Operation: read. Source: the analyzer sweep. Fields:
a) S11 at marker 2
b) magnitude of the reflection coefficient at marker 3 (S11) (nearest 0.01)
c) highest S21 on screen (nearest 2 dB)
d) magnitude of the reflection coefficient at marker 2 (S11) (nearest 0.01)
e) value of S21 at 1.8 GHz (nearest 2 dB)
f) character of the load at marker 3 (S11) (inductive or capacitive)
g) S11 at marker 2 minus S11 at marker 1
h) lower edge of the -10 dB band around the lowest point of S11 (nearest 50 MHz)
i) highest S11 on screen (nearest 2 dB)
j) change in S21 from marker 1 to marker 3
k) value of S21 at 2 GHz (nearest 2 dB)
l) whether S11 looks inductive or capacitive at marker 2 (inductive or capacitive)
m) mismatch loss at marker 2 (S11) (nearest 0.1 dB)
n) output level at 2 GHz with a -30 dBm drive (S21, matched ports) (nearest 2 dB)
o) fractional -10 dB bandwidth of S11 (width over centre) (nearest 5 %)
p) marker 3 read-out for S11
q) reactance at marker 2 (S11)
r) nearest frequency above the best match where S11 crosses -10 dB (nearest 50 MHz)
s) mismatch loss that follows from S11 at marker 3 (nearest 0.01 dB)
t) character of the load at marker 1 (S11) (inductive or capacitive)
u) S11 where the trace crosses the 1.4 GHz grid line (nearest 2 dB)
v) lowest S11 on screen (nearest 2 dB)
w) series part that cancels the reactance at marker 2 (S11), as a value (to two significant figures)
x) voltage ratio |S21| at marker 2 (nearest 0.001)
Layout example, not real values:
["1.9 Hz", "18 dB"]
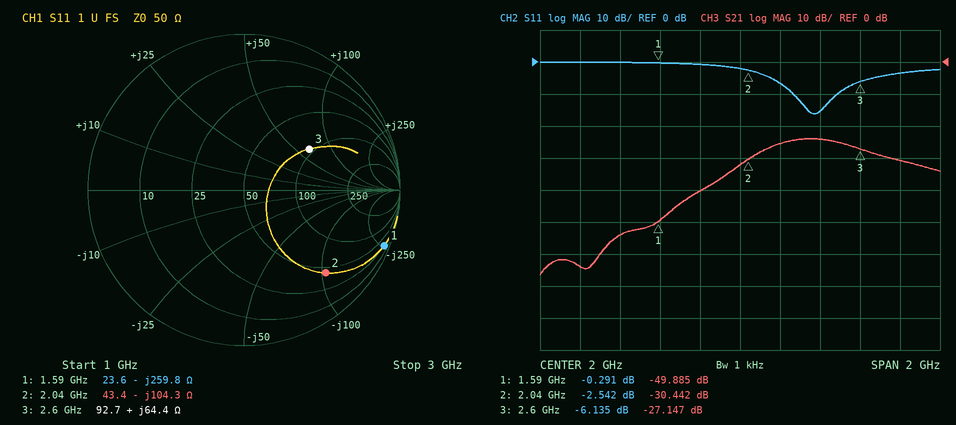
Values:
["-2.542 dB", "0.49", "-24 dB", "0.75", "-40 dB", "inductive", "-2.251 dB", "2.25 GHz", "0 dB", "22.738 dB", "-32 dB", "capacitive", "3.5 dB", "-62 dBm", "10 %", "-6.135 dB", "-104.3 Ω", "2.50 GHz", "1.21 dB", "capacitive", "0 dB", "-16 dB", "8.1 nH", "0.030"]
